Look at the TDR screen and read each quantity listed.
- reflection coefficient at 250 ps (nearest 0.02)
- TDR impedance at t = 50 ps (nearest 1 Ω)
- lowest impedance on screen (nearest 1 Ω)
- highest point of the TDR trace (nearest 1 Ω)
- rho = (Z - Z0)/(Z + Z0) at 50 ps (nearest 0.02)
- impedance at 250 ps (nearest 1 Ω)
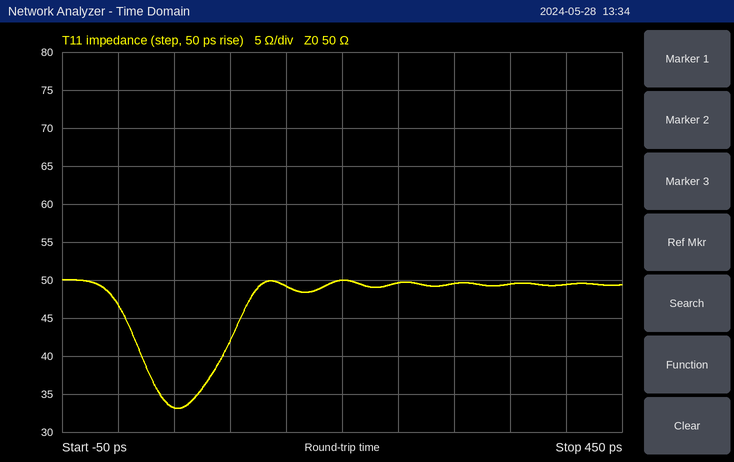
0.00
33 Ω
33 Ω
50 Ω
-0.20
50 Ω
